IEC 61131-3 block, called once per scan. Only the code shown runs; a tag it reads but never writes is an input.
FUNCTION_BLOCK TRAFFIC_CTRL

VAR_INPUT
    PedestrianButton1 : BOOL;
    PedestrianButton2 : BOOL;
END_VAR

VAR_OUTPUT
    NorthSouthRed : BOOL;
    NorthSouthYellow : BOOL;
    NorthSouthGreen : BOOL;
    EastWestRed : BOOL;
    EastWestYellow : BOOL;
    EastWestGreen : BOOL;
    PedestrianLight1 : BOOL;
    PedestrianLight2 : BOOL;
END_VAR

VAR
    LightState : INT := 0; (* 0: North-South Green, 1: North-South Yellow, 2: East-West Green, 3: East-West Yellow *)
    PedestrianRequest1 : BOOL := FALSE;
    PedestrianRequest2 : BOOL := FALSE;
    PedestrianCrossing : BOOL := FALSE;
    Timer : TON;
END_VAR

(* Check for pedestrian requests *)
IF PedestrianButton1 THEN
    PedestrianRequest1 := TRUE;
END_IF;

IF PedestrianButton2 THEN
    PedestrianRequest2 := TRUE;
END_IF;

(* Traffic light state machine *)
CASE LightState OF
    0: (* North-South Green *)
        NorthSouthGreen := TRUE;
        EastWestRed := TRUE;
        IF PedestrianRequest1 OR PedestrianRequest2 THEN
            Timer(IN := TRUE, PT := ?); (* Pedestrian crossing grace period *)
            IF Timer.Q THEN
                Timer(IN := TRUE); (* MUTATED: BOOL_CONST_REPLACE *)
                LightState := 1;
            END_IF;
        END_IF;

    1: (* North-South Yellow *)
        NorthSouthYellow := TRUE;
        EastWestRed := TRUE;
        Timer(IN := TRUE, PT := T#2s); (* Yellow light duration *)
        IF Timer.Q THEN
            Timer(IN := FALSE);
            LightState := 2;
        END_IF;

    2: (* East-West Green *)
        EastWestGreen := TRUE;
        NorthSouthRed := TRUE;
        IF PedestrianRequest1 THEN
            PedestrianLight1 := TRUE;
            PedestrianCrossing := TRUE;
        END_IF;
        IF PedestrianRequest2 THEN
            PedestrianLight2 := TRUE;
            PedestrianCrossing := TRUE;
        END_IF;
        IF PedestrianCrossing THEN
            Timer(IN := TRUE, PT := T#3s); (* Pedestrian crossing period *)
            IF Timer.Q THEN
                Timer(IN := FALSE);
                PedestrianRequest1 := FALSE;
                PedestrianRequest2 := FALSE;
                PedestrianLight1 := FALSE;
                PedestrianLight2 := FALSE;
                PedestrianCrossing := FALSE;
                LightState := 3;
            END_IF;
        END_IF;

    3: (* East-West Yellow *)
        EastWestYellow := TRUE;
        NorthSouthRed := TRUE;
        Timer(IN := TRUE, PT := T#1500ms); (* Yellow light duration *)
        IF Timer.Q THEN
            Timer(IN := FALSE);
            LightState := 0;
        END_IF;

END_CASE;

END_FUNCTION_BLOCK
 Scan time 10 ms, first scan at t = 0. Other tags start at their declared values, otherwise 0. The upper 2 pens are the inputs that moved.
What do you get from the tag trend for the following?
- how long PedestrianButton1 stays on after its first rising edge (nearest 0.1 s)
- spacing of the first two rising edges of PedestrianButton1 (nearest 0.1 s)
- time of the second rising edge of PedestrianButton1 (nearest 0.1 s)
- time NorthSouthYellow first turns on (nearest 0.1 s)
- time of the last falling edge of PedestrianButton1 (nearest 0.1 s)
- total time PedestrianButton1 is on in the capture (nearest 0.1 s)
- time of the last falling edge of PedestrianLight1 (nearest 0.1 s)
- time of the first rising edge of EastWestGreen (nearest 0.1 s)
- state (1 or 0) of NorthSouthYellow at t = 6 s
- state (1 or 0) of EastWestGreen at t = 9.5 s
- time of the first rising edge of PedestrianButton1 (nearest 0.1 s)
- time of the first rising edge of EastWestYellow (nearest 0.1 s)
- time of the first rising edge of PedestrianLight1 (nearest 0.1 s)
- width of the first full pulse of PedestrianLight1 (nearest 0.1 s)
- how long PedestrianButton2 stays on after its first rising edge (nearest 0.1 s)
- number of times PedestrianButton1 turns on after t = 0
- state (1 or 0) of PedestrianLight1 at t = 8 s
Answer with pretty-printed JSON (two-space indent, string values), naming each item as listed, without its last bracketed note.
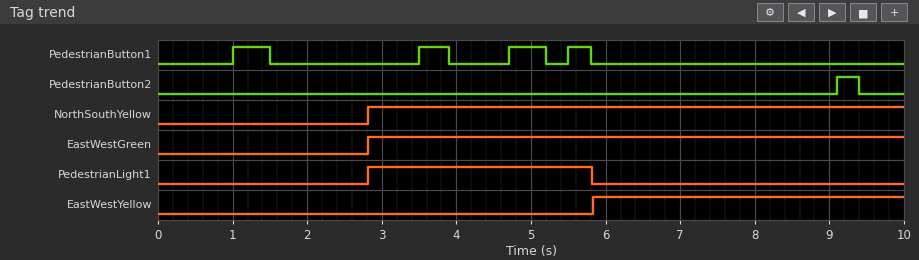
{
  "how long PedestrianButton1 stays on after its first rising edge": "0.5 s",
  "spacing of the first two rising edges of PedestrianButton1": "2.5 s",
  "time of the second rising edge of PedestrianButton1": "3.5 s",
  "time NorthSouthYellow first turns on": "2.8 s",
  "time of the last falling edge of PedestrianButton1": "5.8 s",
  "total time PedestrianButton1 is on in the capture": "1.7 s",
  "time of the last falling edge of PedestrianLight1": "5.8 s",
  "time of the first rising edge of EastWestGreen": "2.8 s",
  "state (1 or 0) of NorthSouthYellow at t = 6 s": "1",
  "state (1 or 0) of EastWestGreen at t = 9.5 s": "1",
  "time of the first rising edge of PedestrianButton1": "1.0 s",
  "time of the first rising edge of EastWestYellow": "5.8 s",
  "time of the first rising edge of PedestrianLight1": "2.8 s",
  "width of the first full pulse of PedestrianLight1": "3.0 s",
  "how long PedestrianButton2 stays on after its first rising edge": "0.3 s",
  "number of times PedestrianButton1 turns on after t = 0": "4",
  "state (1 or 0) of PedestrianLight1 at t = 8 s": "0"
}
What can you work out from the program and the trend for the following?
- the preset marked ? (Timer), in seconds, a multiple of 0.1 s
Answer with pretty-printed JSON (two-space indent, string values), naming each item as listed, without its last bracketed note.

{
  "the preset marked ? (Timer), in seconds, a multiple of 0.1 s": "1.8 s"
}
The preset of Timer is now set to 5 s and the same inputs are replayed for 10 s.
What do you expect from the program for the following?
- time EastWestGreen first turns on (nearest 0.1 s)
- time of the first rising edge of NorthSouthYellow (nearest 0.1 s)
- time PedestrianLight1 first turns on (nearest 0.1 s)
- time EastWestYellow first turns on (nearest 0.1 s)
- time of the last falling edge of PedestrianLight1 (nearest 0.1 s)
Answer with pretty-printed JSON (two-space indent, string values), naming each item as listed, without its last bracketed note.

{
  "time EastWestGreen first turns on": "6.0 s",
  "time of the first rising edge of NorthSouthYellow": "6.0 s",
  "time PedestrianLight1 first turns on": "6.0 s",
  "time EastWestYellow first turns on": "9.0 s",
  "time of the last falling edge of PedestrianLight1": "9.0 s"
}
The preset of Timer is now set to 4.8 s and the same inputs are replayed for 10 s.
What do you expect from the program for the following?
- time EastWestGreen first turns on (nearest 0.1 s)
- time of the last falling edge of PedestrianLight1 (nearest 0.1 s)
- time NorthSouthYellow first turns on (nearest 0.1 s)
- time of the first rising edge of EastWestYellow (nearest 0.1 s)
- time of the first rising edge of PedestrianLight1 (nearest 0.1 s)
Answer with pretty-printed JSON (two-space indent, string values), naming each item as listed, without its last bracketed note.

{
  "time EastWestGreen first turns on": "5.8 s",
  "time of the last falling edge of PedestrianLight1": "8.8 s",
  "time NorthSouthYellow first turns on": "5.8 s",
  "time of the first rising edge of EastWestYellow": "8.8 s",
  "time of the first rising edge of PedestrianLight1": "5.8 s"
}
